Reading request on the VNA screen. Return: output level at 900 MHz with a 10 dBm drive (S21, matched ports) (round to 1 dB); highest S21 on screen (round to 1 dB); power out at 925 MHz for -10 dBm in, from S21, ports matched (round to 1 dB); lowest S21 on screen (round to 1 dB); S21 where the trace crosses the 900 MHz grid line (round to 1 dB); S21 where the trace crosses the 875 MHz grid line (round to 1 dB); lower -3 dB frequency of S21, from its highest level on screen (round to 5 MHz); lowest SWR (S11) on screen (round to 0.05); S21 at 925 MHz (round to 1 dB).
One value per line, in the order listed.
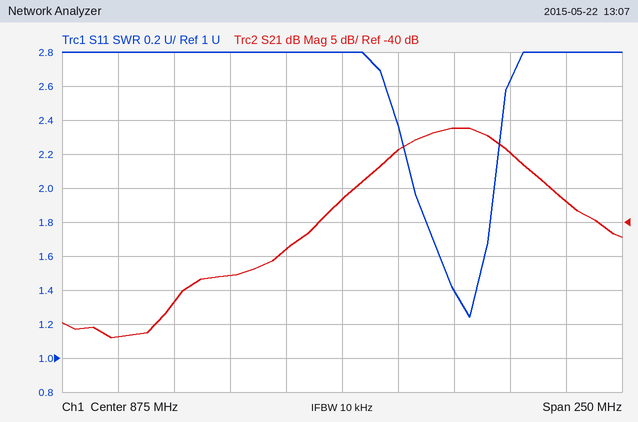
-19 dBm
-26 dB
-36 dBm
-57 dB
-29 dB
-37 dB
900 MHz
1.25
-26 dB
